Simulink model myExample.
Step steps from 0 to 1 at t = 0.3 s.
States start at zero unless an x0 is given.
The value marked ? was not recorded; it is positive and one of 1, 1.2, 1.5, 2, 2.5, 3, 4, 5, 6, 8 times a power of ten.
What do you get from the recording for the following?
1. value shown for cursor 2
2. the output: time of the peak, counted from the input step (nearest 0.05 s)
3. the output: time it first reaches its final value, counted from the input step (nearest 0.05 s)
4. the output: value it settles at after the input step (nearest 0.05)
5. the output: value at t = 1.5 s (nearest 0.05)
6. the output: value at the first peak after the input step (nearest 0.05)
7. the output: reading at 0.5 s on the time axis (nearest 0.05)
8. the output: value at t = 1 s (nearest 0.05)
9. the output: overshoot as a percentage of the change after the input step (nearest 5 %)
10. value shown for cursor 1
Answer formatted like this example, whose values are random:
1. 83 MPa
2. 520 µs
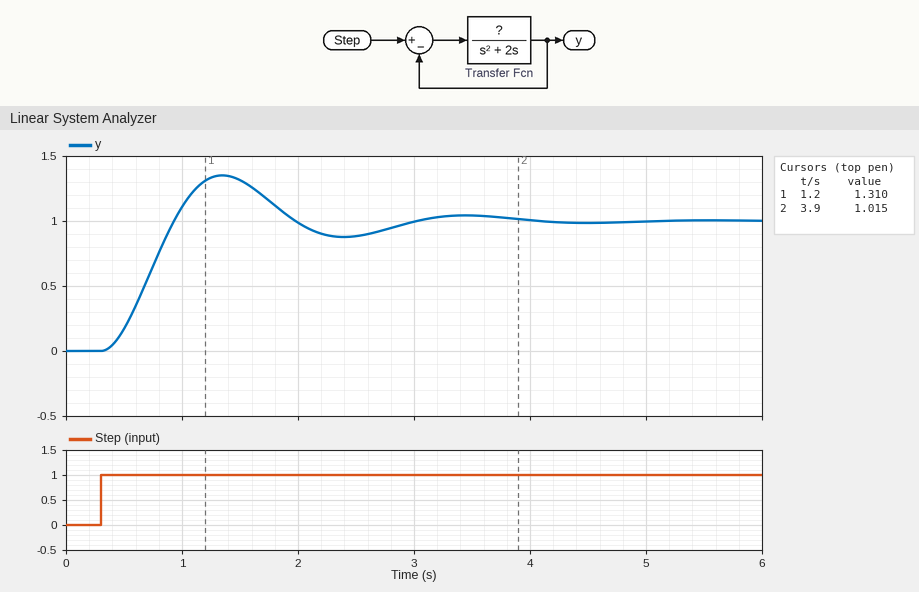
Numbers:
1. 1.015
2. 1.05 s
3. 0.65 s
4. 1.00
5. 1.30
6. 1.35
7. 0.15
8. 1.10
9. 35 %
10. 1.310
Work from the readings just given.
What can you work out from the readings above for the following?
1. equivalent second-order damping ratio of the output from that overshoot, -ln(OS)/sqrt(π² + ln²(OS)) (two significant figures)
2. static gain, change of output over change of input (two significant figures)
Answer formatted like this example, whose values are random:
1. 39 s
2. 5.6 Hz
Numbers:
1. 0.32
2. 1.0
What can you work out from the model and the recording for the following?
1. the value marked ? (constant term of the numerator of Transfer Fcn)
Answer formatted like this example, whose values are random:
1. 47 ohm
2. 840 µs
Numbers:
1. 10
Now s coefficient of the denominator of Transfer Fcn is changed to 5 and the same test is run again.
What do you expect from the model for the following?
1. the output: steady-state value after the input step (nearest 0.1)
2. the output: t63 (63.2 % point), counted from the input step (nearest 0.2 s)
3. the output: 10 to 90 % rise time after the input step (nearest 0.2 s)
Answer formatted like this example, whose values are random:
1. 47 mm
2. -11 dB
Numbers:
1. 1.0
2. 0.6 s
3. 0.8 s
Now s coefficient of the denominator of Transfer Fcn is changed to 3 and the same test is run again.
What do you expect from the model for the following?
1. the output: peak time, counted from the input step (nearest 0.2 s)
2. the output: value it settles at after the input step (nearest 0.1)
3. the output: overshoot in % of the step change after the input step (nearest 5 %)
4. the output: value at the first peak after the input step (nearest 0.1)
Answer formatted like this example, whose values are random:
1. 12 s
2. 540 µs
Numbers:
1. 1.2 s
2. 1.0
3. 20 %
4. 1.2
